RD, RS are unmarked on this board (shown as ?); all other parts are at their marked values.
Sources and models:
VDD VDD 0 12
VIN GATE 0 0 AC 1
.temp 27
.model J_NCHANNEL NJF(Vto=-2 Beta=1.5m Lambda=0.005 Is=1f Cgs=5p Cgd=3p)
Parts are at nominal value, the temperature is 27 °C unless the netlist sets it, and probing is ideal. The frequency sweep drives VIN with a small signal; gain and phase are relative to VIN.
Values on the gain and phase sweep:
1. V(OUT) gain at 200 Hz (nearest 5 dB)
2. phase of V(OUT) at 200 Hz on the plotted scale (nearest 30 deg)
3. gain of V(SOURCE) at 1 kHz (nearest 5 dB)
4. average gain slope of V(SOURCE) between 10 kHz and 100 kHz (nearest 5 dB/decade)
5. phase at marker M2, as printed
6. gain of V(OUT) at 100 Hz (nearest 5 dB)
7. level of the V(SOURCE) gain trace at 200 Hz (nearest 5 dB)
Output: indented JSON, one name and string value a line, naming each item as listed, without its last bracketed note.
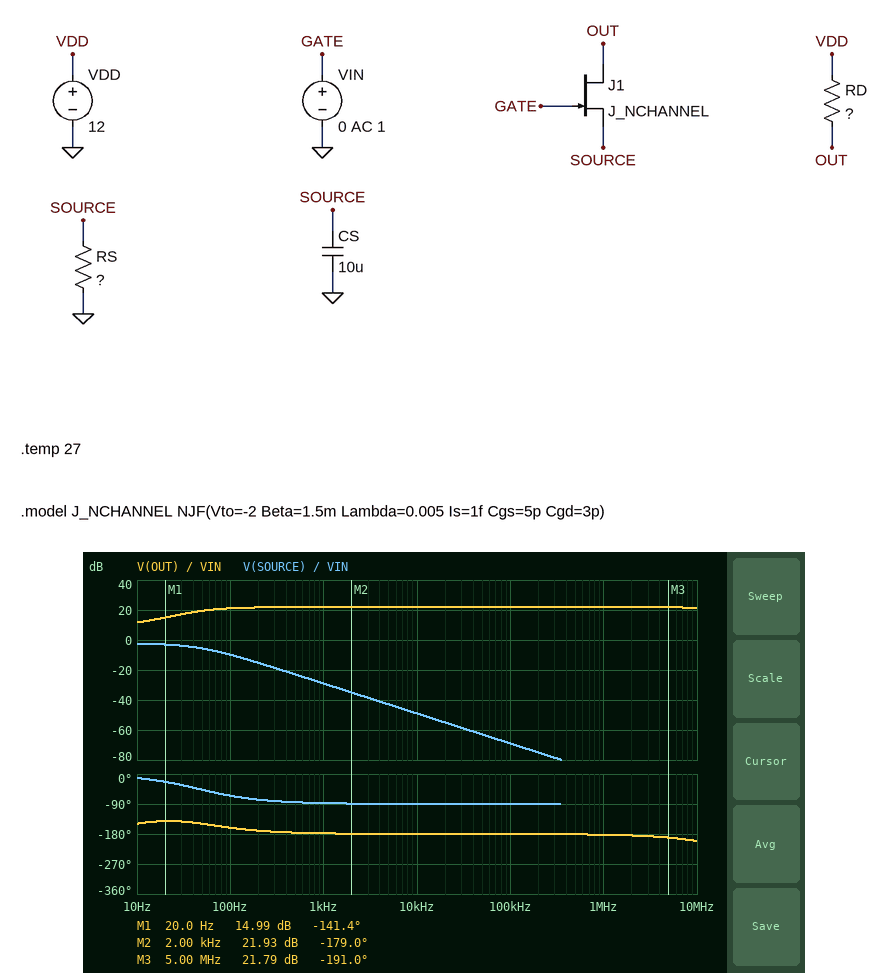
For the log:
{
  "V(OUT) gain at 200 Hz": "20 dB",
  "phase of V(OUT) at 200 Hz on the plotted scale": "-180 deg",
  "gain of V(SOURCE) at 1 kHz": "-30 dB",
  "average gain slope of V(SOURCE) between 10 kHz and 100 kHz": "-20 dB/decade",
  "phase at marker M2, as printed": "-179.0 deg",
  "gain of V(OUT) at 100 Hz": "20 dB",
  "level of the V(SOURCE) gain trace at 200 Hz": "-15 dB"
}
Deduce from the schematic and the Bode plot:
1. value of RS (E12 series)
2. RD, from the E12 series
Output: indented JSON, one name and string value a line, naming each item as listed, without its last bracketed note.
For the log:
{
  "value of RS": "1.5 kΩ",
  "RD, from the E12 series": "5.6 kΩ"
}
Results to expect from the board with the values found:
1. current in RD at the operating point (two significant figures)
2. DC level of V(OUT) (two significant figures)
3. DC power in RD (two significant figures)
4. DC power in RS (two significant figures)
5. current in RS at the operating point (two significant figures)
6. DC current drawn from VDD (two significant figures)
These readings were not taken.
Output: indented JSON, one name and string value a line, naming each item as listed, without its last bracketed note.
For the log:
{
  "current in RD at the operating point": "840 µA",
  "DC level of V(OUT)": "7.3 V",
  "DC power in RD": "4.0 mW",
  "DC power in RS": "1.1 mW",
  "current in RS at the operating point": "840 µA",
  "DC current drawn from VDD": "840 µA"
}
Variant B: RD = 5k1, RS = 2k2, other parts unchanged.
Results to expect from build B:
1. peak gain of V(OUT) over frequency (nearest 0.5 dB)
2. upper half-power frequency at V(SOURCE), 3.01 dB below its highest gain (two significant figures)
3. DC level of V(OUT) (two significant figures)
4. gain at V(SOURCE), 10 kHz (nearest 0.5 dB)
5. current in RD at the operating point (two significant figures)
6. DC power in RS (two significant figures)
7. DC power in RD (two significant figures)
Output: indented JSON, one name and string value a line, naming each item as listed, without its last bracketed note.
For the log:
{
  "peak gain of V(OUT) over frequency": "20.0 dB",
  "upper half-power frequency at V(SOURCE), 3.01 dB below its highest gain": "38 Hz",
  "DC level of V(OUT)": "8.8 V",
  "gain at V(SOURCE), 10 kHz": "-50.0 dB",
  "current in RD at the operating point": "620 µA",
  "DC power in RS": "850 µW",
  "DC power in RD": "2.0 mW"
}
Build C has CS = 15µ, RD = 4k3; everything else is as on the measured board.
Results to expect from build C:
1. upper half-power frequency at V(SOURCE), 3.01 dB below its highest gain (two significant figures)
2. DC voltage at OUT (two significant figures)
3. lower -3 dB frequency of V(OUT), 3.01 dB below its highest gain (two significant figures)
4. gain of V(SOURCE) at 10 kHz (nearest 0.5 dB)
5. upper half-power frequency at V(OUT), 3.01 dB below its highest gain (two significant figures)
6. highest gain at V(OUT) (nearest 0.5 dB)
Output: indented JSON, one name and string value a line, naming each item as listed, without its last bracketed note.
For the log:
{
  "upper half-power frequency at V(SOURCE), 3.01 dB below its highest gain": "31 Hz",
  "DC voltage at OUT": "8.4 V",
  "lower -3 dB frequency of V(OUT), 3.01 dB below its highest gain": "29 Hz",
  "gain of V(SOURCE) at 10 kHz": "-52.5 dB",
  "upper half-power frequency at V(OUT), 3.01 dB below its highest gain": "39 MHz",
  "highest gain at V(OUT)": "19.5 dB"
}
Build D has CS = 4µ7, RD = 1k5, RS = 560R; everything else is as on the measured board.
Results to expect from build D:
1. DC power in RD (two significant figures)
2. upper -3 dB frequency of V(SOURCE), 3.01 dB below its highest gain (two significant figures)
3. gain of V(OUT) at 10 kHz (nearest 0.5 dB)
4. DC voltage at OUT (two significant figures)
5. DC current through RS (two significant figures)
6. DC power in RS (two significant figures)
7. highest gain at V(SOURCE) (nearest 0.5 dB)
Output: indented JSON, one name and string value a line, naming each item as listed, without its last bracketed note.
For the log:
{
  "DC power in RD": "4.4 mW",
  "upper -3 dB frequency of V(SOURCE), 3.01 dB below its highest gain": "170 Hz",
  "gain of V(OUT) at 10 kHz": "13.5 dB",
  "DC voltage at OUT": "9.4 V",
  "DC current through RS": "1.7 mA",
  "DC power in RS": "1.6 mW",
  "highest gain at V(SOURCE)": "-4.0 dB"
}
